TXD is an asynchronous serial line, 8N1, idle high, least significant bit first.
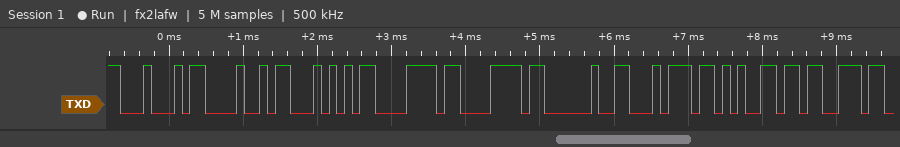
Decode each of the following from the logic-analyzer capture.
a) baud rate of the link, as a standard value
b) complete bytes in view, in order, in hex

9600 baud
0x44 0x48 0x54 0x78 0x78 0x20 0x74 0x65 0x73
